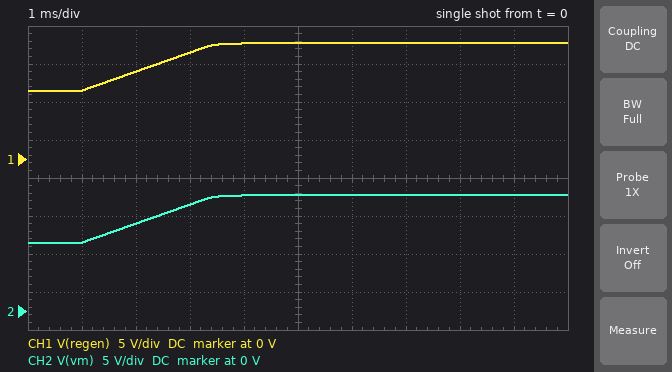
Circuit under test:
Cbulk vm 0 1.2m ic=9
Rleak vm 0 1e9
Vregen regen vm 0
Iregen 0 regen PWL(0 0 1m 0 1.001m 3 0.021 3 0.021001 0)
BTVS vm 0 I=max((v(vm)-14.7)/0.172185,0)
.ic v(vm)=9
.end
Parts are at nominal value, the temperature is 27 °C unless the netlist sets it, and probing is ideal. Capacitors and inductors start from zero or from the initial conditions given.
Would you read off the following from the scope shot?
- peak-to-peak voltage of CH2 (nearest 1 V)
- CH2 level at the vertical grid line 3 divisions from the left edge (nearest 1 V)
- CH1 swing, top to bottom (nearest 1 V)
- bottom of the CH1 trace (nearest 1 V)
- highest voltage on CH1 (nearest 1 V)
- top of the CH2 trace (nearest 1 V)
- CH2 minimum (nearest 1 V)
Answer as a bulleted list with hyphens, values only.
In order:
- 6 V
- 14 V
- 6 V
- 9 V
- 15 V
- 15 V
- 9 V
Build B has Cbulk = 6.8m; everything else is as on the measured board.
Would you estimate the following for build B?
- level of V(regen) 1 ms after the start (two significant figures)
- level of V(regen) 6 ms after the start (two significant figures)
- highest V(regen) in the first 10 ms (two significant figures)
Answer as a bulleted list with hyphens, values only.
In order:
- 9.0 V
- 11 V
- 13 V
